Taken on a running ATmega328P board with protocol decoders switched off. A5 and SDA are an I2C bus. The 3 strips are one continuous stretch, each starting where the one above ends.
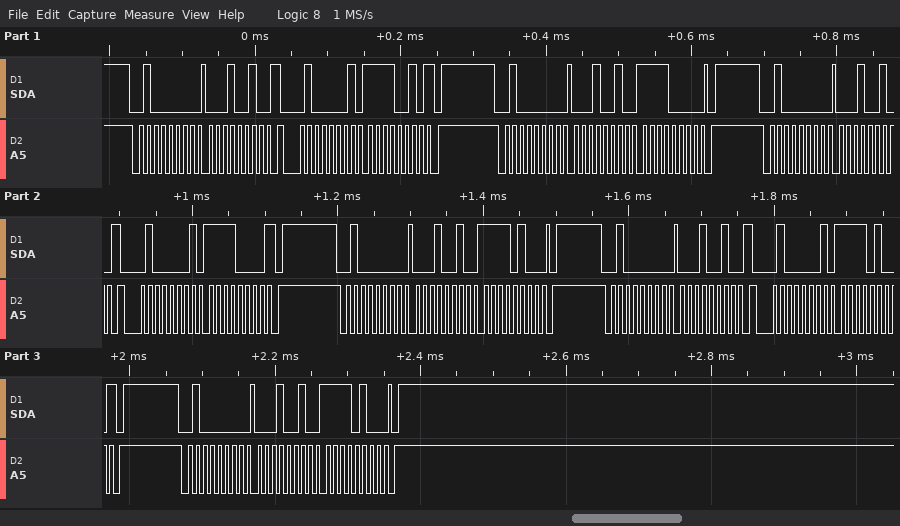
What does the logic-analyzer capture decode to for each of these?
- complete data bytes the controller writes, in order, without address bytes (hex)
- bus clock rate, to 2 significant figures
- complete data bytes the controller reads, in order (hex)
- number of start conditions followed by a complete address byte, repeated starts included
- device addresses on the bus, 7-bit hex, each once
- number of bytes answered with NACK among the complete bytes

12 12 F0 12 12 F4 12 12 F4
100 kHz
F2 F0 F4
9
0x20
3
